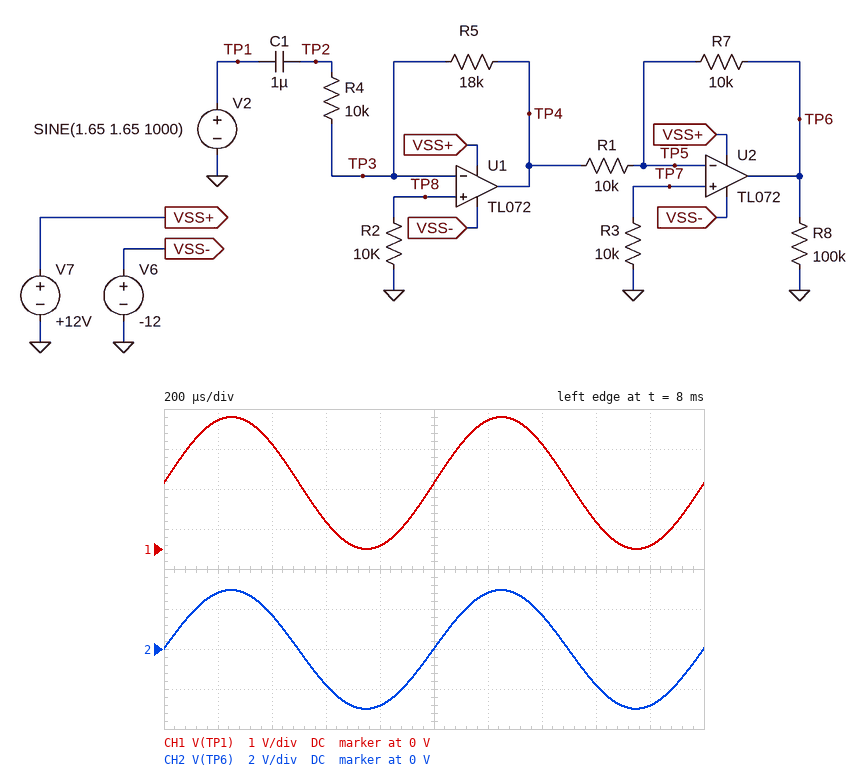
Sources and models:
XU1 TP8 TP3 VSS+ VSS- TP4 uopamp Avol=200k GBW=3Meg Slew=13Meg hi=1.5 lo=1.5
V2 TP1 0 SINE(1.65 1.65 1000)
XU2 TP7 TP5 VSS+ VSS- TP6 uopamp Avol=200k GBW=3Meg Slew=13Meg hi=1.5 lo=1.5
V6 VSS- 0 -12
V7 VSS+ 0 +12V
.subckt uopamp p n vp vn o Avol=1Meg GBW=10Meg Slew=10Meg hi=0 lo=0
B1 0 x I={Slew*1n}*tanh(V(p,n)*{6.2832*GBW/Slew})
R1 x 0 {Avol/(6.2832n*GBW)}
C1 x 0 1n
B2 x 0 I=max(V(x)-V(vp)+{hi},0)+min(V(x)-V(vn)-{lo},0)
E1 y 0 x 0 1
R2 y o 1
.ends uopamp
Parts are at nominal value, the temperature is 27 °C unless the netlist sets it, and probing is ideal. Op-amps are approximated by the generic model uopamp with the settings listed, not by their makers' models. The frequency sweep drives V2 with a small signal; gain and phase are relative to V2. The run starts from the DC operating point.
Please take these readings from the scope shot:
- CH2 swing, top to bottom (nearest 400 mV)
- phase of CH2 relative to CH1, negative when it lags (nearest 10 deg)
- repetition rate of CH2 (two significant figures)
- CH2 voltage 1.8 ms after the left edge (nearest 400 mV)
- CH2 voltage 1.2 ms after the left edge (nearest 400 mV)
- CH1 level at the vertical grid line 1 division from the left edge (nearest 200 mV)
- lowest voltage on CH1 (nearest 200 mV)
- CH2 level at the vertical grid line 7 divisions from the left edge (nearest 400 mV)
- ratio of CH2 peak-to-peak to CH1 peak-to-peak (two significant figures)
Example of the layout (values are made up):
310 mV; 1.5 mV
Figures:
6.0 V; 0 deg; 1.0 kHz; -2.8 V; 2.8 V; 3.2 V; 0 V; 1.6 V; 1.8
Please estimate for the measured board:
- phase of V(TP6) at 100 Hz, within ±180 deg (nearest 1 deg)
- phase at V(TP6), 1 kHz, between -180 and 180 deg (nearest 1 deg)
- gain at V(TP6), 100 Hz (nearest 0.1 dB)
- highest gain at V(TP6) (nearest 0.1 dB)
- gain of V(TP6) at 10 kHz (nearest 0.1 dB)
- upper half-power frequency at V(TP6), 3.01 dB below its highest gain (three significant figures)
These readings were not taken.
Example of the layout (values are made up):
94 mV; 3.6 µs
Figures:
9 deg; 1 deg; 5.0 dB; 5.1 dB; 5.1 dB; 800 kHz
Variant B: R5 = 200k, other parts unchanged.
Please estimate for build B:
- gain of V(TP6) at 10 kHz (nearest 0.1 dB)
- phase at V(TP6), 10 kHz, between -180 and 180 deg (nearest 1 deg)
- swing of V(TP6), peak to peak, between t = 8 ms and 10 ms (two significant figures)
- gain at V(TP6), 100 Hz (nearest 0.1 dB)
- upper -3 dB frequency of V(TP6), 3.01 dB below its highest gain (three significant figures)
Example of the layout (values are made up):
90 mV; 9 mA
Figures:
26.0 dB; -4 deg; 21 V; 25.9 dB; 142 kHz
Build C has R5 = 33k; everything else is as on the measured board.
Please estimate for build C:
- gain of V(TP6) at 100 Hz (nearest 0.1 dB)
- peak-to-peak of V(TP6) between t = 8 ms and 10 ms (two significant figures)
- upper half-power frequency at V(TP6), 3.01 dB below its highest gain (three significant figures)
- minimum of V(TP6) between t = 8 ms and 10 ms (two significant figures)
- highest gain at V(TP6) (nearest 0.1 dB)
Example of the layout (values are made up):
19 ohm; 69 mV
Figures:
10.3 dB; 11 V; 595 kHz; -5.5 V; 10.4 dB
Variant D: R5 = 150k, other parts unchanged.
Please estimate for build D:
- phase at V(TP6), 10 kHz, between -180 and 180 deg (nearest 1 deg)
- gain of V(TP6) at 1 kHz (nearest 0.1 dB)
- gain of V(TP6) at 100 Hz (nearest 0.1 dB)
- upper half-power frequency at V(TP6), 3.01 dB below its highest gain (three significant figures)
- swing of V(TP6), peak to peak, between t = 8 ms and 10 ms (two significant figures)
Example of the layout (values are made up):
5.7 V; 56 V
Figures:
-3 deg; 23.5 dB; 23.4 dB; 185 kHz; 21 V
